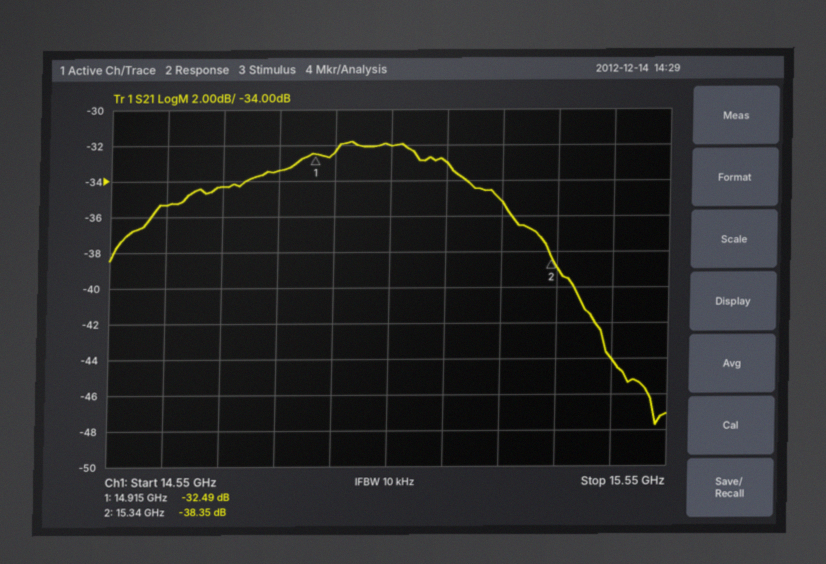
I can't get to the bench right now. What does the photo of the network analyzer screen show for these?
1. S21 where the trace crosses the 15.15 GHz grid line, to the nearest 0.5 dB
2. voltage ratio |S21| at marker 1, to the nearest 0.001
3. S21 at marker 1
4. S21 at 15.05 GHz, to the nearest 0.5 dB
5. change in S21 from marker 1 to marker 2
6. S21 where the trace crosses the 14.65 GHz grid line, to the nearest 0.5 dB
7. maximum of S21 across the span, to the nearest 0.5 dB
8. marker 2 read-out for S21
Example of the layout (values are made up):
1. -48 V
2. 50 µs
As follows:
1. -33.0 dB
2. 0.024
3. -32.49 dB
4. -32.0 dB
5. -5.86 dB
6. -35.5 dB
7. -32.0 dB
8. -38.35 dB
